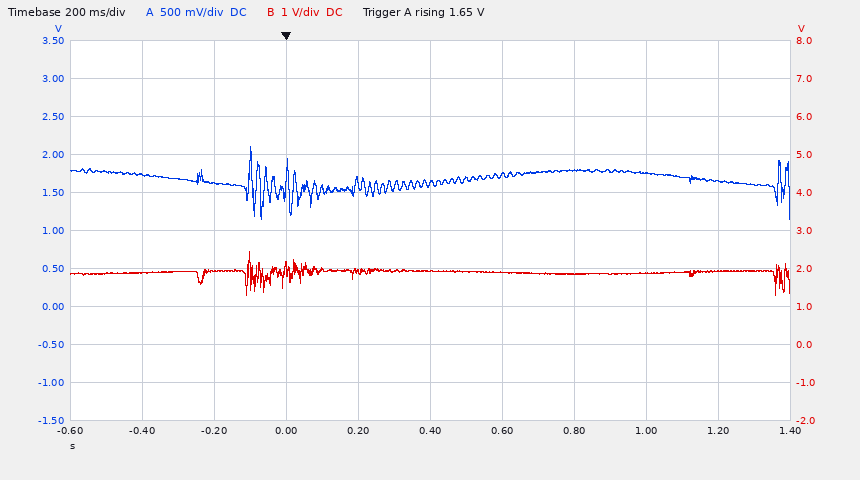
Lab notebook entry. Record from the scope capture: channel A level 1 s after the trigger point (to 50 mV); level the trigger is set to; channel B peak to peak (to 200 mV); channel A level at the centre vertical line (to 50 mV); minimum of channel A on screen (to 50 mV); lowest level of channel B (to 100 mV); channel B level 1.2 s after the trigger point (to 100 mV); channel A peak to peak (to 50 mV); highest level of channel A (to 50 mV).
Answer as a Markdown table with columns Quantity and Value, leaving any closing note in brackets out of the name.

| Quantity | Value |
|---|---|
| channel A level 1 s after the trigger point | 1.75 V |
| level the trigger is set to | 1.65 V |
| channel B peak to peak | 1.2 V |
| channel A level at the centre vertical line | 1.60 V |
| minimum of channel A on screen | 1.15 V |
| lowest level of channel B | 1.3 V |
| channel B level 1.2 s after the trigger point | 1.9 V |
| channel A peak to peak | 950 mV |
| highest level of channel A | 2.10 V |
